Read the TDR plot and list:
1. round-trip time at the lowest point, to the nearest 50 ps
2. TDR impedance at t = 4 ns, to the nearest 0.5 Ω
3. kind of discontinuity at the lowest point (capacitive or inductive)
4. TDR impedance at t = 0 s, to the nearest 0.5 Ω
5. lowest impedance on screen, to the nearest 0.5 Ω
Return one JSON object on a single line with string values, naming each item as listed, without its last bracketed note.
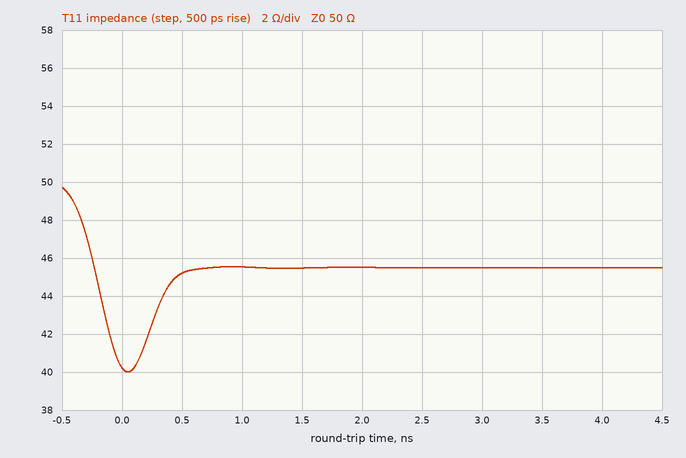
{"round-trip time at the lowest point, to the nearest 50 ps": "50 ps", "TDR impedance at t = 4 ns, to the nearest 0.5 Ω": "45.5 Ω", "kind of discontinuity at the lowest point": "capacitive", "TDR impedance at t = 0 s, to the nearest 0.5 Ω": "40.0 Ω", "lowest impedance on screen, to the nearest 0.5 Ω": "40.0 Ω"}
